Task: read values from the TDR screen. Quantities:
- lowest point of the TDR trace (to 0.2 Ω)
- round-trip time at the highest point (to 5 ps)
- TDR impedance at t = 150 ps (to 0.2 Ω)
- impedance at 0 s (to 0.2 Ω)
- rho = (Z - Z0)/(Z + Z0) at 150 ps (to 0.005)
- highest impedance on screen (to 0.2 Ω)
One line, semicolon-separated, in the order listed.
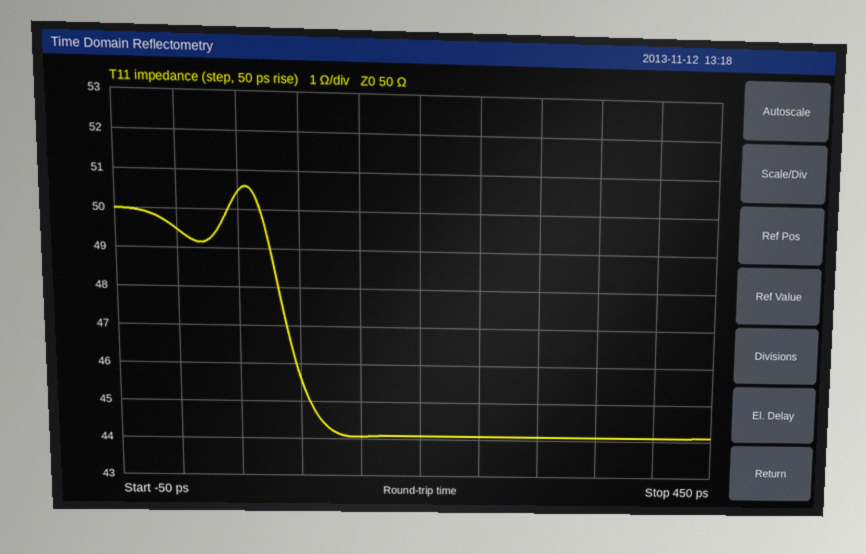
44.0 Ω; 55 ps; 44.0 Ω; 49.4 Ω; -0.065; 50.6 Ω
